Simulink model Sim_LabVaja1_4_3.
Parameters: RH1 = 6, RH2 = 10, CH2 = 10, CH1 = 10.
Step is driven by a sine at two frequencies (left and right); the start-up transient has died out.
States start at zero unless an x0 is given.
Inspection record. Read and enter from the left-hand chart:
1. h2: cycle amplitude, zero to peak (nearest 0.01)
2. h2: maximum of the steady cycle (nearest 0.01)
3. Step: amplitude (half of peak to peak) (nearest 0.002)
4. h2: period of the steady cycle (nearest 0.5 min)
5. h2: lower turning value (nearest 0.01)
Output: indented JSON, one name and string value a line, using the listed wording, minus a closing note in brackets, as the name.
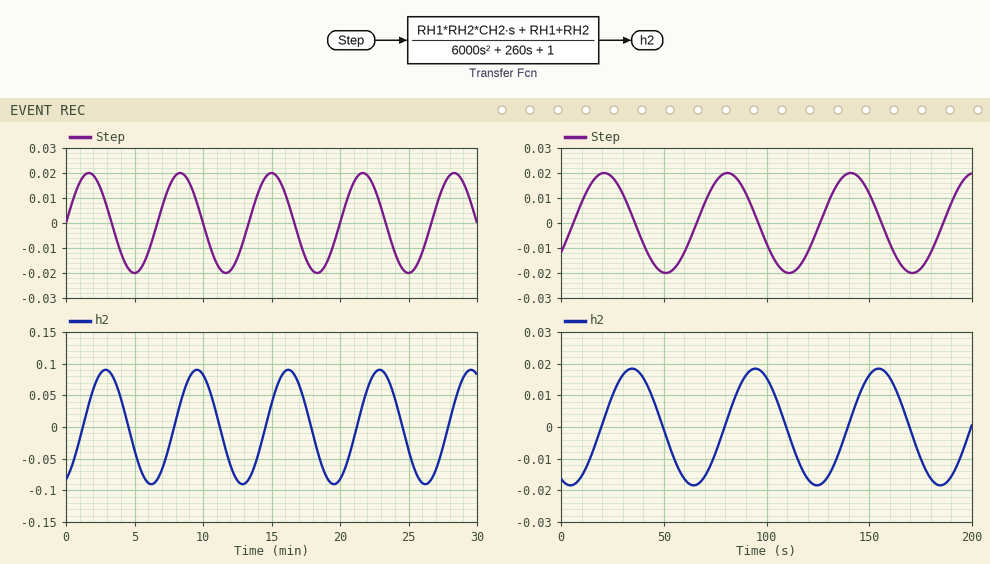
{
  "h2: cycle amplitude, zero to peak": "0.09",
  "h2: maximum of the steady cycle": "0.09",
  "Step: amplitude (half of peak to peak)": "0.020",
  "h2: period of the steady cycle": "6.5 min",
  "h2: lower turning value": "-0.09"
}
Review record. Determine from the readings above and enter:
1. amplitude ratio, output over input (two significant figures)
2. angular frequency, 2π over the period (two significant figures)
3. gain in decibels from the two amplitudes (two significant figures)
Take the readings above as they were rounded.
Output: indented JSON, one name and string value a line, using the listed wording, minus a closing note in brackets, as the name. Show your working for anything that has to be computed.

{
  "amplitude ratio, output over input": "0.09 / 0.02 = 4.5",
  "angular frequency, 2π over the period": "2π / 6.5 = 0.97 rad/min",
  "gain in decibels from the two amplitudes": "20 log10(0.09 / 0.02) = 13 dB"
}
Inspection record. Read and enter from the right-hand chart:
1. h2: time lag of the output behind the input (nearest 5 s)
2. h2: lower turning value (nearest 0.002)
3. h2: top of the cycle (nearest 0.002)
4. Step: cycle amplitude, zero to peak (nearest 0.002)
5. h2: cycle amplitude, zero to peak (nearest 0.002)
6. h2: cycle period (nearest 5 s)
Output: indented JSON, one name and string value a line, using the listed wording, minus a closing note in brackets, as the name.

{
  "h2: time lag of the output behind the input": "15 s",
  "h2: lower turning value": "-0.018",
  "h2: top of the cycle": "0.018",
  "Step: cycle amplitude, zero to peak": "0.020",
  "h2: cycle amplitude, zero to peak": "0.018",
  "h2: cycle period": "60 s"
}
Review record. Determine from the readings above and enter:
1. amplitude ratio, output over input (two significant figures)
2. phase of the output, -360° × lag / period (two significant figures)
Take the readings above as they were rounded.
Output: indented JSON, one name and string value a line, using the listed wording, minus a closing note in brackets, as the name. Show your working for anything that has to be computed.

{
  "amplitude ratio, output over input": "0.018 / 0.02 = 0.90",
  "phase of the output, -360° × lag / period": "-360 × 15 / 60 = -90°"
}
